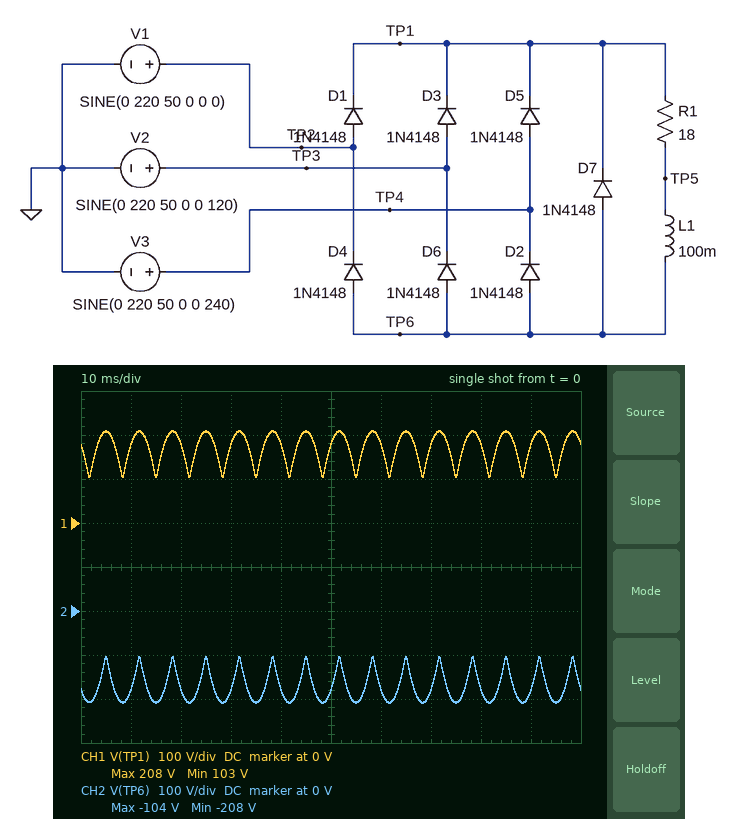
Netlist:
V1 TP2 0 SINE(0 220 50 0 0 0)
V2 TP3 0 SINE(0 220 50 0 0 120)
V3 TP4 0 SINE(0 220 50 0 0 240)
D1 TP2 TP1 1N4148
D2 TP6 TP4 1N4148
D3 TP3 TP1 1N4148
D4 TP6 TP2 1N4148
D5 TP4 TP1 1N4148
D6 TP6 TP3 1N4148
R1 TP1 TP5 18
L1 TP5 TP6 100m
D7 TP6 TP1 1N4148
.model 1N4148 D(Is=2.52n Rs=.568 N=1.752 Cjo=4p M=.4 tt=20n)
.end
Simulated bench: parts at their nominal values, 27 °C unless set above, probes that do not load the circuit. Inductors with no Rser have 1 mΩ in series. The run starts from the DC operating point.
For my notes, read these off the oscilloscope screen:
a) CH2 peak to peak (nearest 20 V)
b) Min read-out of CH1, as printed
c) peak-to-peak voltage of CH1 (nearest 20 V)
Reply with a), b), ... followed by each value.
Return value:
a) 100 V
b) 103 V
c) 100 V
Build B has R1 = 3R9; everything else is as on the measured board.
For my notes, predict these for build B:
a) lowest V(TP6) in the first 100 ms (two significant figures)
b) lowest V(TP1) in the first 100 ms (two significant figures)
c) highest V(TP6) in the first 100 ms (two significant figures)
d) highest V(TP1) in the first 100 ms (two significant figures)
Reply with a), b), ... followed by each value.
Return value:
a) -180 V
b) 87 V
c) -87 V
d) 180 V
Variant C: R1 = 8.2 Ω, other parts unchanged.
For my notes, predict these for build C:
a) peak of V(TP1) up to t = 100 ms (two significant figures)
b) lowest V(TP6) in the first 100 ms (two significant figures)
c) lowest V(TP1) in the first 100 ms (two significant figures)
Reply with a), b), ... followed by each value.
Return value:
a) 200 V
b) -200 V
c) 97 V
